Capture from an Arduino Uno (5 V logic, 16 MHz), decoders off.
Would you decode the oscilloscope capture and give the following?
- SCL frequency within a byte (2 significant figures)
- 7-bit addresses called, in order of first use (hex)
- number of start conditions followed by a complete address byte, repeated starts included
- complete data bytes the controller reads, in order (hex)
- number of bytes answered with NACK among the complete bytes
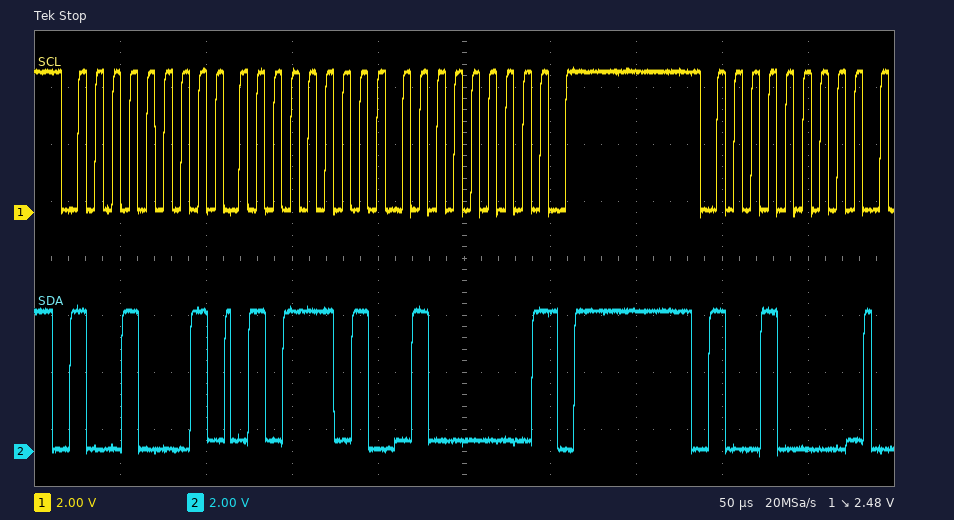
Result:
100 kHz
0x48
2
5D 40
1
